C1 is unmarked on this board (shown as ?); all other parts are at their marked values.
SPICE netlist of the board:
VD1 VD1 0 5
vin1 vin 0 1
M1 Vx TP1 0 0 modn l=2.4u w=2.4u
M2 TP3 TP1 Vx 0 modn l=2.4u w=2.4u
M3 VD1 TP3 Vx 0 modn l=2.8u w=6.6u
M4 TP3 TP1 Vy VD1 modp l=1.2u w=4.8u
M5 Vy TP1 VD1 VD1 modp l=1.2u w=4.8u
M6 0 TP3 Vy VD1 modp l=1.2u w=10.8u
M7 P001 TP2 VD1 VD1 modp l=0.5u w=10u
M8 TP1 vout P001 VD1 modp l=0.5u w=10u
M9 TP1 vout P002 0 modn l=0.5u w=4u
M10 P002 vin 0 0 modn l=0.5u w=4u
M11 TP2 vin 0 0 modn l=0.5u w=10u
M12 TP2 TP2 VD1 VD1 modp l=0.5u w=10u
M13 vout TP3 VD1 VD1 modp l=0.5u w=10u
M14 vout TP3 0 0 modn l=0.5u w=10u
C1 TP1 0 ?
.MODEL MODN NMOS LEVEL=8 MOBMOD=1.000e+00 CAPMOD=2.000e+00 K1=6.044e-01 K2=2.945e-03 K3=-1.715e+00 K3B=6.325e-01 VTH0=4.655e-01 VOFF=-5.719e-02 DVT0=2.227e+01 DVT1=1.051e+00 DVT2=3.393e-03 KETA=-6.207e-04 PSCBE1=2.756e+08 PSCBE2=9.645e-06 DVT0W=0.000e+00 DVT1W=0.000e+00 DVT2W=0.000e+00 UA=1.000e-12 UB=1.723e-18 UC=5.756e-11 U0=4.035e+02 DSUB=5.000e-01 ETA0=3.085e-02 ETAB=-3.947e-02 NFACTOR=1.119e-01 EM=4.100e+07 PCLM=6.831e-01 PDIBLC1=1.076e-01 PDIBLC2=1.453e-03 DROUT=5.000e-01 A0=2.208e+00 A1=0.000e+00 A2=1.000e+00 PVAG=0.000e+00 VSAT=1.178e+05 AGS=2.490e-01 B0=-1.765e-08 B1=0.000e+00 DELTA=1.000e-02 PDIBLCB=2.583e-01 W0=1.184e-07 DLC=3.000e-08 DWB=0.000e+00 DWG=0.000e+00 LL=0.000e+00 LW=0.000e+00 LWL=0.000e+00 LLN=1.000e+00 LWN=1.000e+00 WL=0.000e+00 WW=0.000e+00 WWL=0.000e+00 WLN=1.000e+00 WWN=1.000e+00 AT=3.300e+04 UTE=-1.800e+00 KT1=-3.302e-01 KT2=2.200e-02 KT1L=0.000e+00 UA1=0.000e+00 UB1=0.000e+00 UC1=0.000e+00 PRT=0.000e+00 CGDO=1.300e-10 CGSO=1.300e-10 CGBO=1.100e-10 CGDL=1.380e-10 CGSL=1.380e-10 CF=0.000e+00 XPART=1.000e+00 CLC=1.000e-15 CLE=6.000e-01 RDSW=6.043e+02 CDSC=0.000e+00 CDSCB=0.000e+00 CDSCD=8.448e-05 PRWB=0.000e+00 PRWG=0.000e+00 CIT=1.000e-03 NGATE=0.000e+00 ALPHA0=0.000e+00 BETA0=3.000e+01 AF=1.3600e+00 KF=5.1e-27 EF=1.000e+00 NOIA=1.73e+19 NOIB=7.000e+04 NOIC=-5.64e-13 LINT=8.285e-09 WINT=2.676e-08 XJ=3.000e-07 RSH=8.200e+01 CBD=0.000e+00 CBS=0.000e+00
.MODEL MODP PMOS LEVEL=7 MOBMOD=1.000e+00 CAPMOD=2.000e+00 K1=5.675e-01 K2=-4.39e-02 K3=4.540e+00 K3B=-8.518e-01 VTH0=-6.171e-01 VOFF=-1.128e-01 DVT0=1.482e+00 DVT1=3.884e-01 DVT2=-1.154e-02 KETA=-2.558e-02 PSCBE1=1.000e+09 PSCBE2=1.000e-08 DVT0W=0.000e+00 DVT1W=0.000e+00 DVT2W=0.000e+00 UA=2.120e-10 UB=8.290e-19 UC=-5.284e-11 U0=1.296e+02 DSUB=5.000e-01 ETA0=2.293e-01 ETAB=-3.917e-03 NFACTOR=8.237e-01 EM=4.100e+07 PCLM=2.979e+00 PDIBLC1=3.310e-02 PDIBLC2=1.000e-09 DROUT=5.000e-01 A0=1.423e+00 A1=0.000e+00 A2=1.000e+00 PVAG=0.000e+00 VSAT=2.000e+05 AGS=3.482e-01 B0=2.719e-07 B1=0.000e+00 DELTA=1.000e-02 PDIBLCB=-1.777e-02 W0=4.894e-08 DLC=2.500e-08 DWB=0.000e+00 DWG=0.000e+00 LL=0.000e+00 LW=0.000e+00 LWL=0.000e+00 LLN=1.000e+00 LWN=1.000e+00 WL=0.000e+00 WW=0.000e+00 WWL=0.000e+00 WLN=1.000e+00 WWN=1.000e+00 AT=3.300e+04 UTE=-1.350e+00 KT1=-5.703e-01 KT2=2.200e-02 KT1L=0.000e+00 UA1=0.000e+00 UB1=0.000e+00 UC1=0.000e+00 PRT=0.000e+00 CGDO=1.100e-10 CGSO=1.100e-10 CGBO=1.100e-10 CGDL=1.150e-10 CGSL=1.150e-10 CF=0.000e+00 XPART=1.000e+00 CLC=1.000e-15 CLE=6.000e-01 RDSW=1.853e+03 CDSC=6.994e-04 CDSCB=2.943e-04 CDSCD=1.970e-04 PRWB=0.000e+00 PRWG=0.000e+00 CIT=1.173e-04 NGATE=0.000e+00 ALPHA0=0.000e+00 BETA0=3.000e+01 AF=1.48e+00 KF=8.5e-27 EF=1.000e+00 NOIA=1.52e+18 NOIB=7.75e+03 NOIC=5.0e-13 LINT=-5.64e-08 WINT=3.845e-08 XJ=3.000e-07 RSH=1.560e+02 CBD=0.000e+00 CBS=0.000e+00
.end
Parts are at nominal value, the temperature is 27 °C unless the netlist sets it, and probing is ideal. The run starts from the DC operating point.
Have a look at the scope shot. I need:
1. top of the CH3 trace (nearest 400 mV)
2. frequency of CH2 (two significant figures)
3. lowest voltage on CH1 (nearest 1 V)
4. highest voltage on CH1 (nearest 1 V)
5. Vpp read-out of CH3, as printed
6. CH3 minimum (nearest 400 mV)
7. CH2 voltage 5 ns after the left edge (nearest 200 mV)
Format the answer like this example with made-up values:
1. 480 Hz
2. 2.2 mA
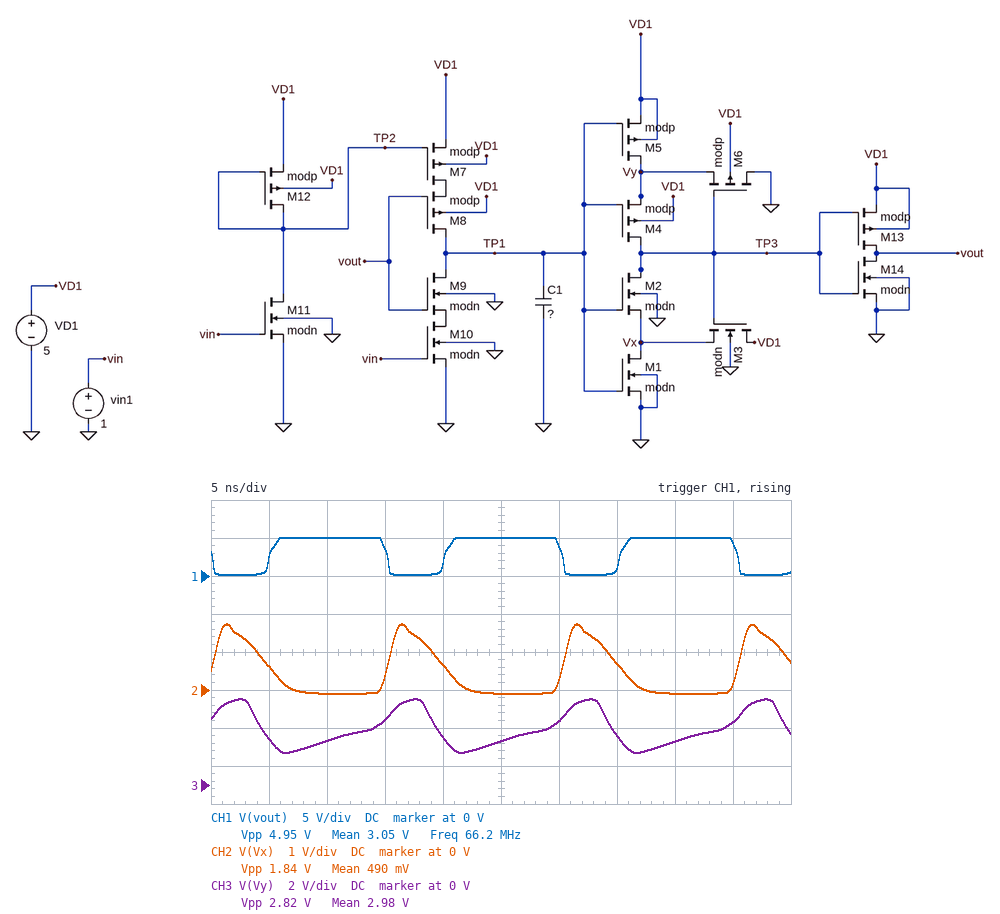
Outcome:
1. 4.4 V
2. 66 MHz
3. 0 V
4. 5 V
5. 2.82 V
6. 1.6 V
7. 600 mV
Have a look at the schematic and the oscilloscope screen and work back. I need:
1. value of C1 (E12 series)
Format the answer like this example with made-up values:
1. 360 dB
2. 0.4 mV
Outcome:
1. 330 fF
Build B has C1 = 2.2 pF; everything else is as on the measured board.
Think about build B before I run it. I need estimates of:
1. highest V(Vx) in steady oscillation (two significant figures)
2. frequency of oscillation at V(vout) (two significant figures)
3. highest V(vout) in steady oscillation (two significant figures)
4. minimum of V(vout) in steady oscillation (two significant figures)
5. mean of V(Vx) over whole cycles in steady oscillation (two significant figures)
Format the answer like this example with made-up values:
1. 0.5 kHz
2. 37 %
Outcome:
1. 2.7 V
2. 18 MHz
3. 5.0 V
4. -1.7 mV
5. 680 mV
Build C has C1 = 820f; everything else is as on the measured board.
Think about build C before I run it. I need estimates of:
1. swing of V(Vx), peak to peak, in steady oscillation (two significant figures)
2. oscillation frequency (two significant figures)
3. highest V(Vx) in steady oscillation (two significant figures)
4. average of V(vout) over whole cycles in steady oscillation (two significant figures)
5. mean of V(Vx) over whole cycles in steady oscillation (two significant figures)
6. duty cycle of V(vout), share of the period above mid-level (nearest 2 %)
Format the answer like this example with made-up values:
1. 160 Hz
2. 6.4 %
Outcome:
1. 2.2 V
2. 36 MHz
3. 2.1 V
4. 3.3 V
5. 560 mV
6. 66 %
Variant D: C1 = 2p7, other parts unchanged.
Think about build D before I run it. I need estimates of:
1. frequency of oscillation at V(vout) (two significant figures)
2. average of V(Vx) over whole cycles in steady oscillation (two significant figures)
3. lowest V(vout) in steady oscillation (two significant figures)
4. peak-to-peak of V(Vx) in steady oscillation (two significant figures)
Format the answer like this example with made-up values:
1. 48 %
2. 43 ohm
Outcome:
1. 15 MHz
2. 700 mV
3. -1.7 mV
4. 2.8 V
